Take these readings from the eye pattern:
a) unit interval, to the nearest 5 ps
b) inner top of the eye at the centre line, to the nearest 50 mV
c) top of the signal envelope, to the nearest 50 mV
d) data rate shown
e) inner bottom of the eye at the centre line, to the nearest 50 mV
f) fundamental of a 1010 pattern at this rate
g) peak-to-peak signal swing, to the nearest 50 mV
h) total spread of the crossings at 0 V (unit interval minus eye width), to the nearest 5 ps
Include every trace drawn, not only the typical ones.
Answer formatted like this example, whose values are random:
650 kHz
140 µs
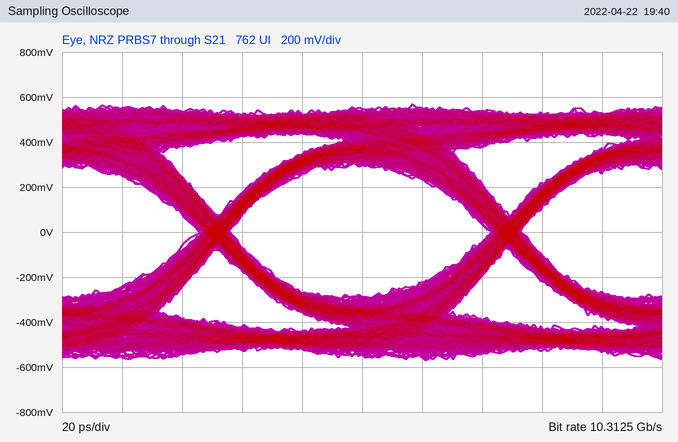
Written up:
95 ps
300 mV
550 mV
10.3125 Gb/s
-300 mV
5.15625 GHz
1.15 V
10 ps
